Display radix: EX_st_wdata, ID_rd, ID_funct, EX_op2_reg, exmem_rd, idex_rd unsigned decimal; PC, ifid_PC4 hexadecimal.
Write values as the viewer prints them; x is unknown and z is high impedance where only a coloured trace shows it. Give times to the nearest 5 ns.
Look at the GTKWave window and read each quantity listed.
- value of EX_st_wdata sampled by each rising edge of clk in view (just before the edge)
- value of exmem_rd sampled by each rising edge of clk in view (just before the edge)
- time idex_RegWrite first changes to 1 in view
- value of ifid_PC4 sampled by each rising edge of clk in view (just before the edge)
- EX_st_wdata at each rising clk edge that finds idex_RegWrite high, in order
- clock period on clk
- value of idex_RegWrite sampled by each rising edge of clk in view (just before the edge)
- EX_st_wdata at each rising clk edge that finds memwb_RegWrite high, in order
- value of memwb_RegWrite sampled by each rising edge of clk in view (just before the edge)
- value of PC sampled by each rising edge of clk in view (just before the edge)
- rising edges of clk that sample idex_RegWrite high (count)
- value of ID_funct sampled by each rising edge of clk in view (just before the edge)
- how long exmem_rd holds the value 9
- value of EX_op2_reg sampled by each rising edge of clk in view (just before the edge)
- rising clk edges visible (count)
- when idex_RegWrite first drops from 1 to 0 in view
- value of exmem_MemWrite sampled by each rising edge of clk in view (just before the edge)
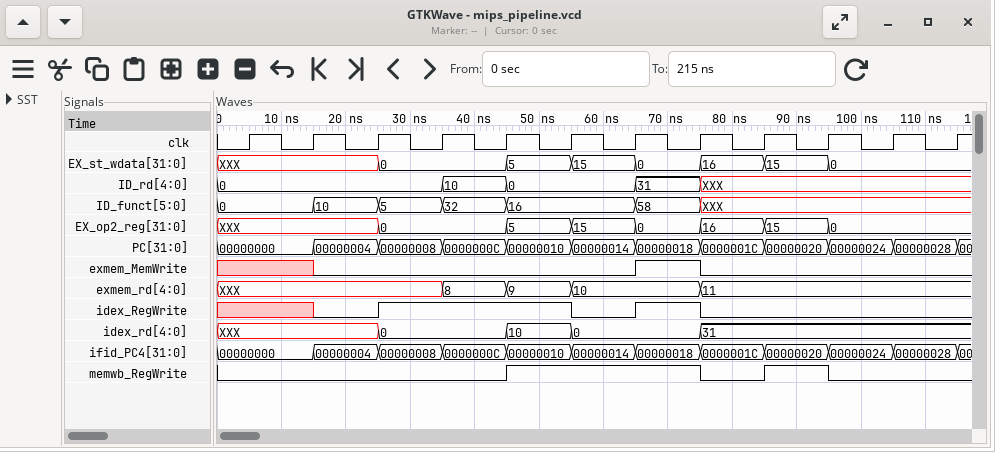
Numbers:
XXX, XXX, XXX, 0, 0, 5, 15, 0, 16, 15, 0, 0
XXX, XXX, XXX, XXX, 8, 9, 10, 10, 11, 11, 11, 11
25 ns
00000000, 00000000, 00000004, 00000008, 0000000C, 00000010, 00000014, 00000018, 0000001C, 00000020, 00000024, 00000028
0, 0, 5, 0
10 ns
x x 0 1 1 1 0 1 0 0 0 0
5, 15, 0, 15
0 0 0 0 0 1 1 1 0 1 0 0
00000000, 00000000, 00000004, 00000008, 0000000C, 00000010, 00000014, 00000018, 0000001C, 00000020, 00000024, 00000028
4
0, 0, 10, 5, 32, 16, 16, 58, XXX, XXX, XXX, XXX
10 ns
XXX, XXX, XXX, 0, 0, 5, 15, 0, 16, 15, 0, 0
12
55 ns
x x 0 0 0 0 0 1 0 0 0 0
